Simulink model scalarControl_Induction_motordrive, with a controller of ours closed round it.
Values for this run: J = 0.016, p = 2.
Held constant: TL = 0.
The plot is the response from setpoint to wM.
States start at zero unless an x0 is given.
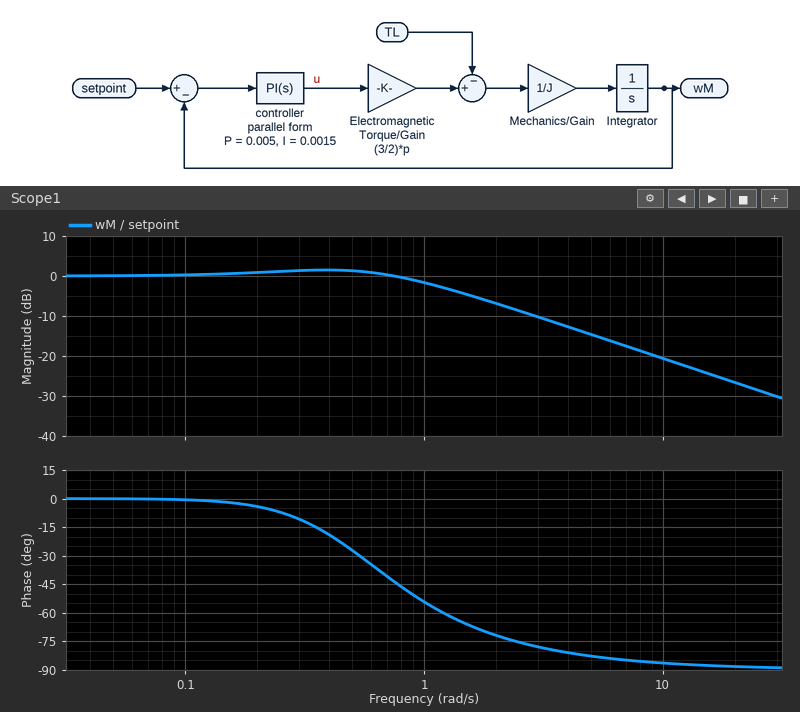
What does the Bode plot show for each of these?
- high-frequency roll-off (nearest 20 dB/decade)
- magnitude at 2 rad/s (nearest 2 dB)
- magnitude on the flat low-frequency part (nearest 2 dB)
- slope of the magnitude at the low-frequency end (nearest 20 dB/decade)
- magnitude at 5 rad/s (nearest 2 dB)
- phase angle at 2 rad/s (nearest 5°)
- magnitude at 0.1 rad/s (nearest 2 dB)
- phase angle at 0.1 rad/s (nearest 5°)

-20 dB/decade
-6 dB
0 dB
0 dB/decade
-14 dB
-70°
0 dB
0°
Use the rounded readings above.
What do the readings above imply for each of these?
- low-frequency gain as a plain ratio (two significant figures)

1.0
